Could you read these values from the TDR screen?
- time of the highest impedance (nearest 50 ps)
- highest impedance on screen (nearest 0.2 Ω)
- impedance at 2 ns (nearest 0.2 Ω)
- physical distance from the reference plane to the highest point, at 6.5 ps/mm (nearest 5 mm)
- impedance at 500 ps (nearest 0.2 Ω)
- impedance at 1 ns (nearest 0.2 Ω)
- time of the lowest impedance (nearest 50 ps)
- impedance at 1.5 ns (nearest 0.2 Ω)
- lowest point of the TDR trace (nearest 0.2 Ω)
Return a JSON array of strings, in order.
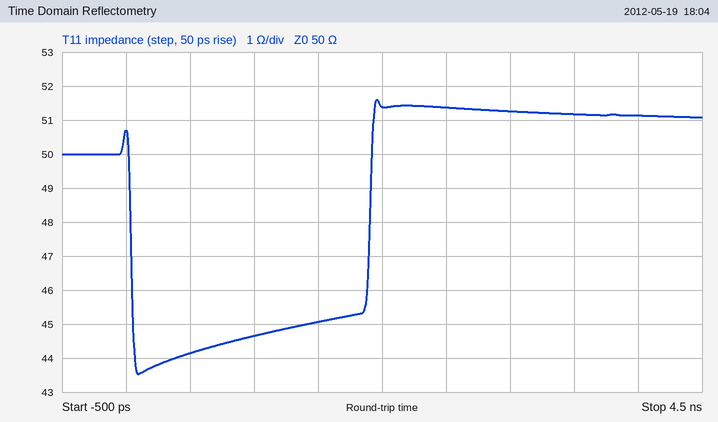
["1.95 ns", "51.6 Ω", "51.4 Ω", "150 mm", "44.2 Ω", "44.6 Ω", "100 ps", "45.0 Ω", "43.6 Ω"]
